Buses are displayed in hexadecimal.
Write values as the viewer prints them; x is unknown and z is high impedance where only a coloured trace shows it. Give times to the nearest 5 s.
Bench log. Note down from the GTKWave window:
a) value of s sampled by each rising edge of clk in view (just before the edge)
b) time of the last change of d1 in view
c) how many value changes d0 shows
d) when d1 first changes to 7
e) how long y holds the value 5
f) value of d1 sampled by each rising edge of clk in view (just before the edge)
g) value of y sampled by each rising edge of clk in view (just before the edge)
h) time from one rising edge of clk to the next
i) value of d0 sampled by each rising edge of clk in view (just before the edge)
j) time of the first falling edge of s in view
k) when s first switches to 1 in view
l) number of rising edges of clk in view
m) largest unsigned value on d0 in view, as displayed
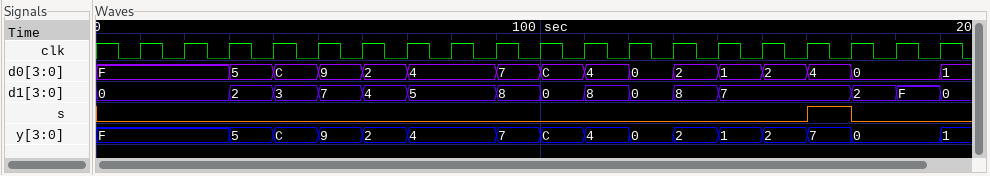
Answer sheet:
0 0 0 0 0 0 0 0 0 0 0 0 0 0 0 0 1 0 0
190 s
15
50 s
10 s
0, 0, 0, 2, 3, 7, 4, 5, 5, 8, 0, 8, 0, 8, 7, 7, 7, 2, F
F, F, F, 5, C, 9, 2, 4, 4, 7, C, 4, 0, 2, 1, 2, 7, 0, 0
10 s
F, F, F, 5, C, 9, 2, 4, 4, 7, C, 4, 0, 2, 1, 2, 4, 0, 0
170 s
160 s
19
F
